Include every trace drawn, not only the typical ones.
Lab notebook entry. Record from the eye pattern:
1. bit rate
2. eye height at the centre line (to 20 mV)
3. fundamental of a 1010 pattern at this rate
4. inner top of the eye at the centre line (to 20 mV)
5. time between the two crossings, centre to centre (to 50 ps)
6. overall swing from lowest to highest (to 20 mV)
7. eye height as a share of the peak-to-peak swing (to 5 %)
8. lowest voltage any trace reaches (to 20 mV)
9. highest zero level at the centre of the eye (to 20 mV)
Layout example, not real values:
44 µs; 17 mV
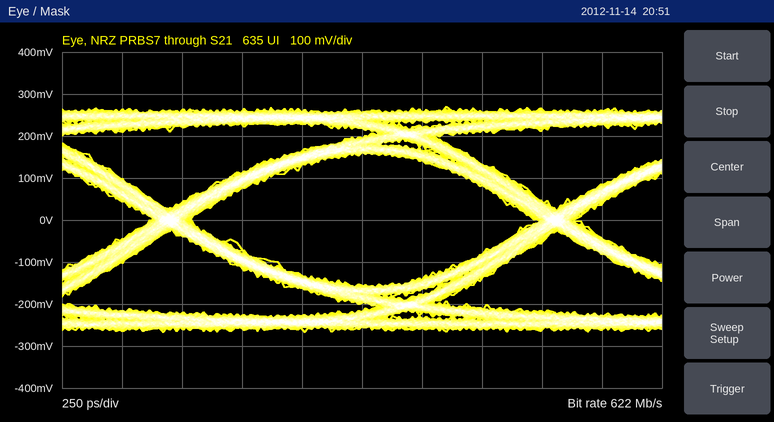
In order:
622 Mb/s; 320 mV; 311 MHz; 160 mV; 1.60 ns; 540 mV; 60 %; -260 mV; -160 mV
